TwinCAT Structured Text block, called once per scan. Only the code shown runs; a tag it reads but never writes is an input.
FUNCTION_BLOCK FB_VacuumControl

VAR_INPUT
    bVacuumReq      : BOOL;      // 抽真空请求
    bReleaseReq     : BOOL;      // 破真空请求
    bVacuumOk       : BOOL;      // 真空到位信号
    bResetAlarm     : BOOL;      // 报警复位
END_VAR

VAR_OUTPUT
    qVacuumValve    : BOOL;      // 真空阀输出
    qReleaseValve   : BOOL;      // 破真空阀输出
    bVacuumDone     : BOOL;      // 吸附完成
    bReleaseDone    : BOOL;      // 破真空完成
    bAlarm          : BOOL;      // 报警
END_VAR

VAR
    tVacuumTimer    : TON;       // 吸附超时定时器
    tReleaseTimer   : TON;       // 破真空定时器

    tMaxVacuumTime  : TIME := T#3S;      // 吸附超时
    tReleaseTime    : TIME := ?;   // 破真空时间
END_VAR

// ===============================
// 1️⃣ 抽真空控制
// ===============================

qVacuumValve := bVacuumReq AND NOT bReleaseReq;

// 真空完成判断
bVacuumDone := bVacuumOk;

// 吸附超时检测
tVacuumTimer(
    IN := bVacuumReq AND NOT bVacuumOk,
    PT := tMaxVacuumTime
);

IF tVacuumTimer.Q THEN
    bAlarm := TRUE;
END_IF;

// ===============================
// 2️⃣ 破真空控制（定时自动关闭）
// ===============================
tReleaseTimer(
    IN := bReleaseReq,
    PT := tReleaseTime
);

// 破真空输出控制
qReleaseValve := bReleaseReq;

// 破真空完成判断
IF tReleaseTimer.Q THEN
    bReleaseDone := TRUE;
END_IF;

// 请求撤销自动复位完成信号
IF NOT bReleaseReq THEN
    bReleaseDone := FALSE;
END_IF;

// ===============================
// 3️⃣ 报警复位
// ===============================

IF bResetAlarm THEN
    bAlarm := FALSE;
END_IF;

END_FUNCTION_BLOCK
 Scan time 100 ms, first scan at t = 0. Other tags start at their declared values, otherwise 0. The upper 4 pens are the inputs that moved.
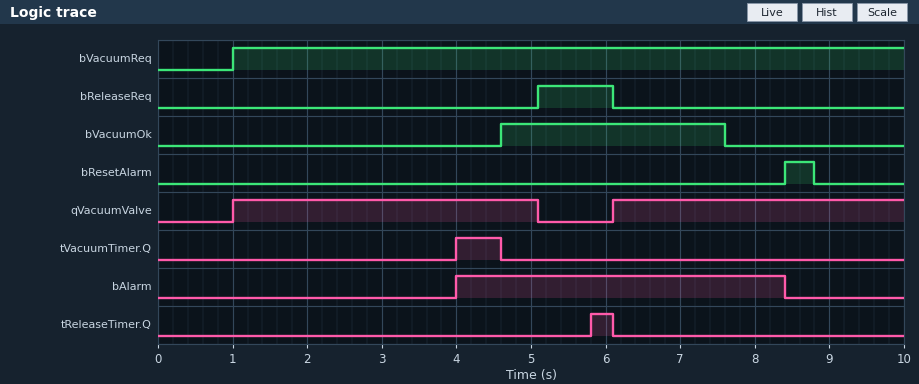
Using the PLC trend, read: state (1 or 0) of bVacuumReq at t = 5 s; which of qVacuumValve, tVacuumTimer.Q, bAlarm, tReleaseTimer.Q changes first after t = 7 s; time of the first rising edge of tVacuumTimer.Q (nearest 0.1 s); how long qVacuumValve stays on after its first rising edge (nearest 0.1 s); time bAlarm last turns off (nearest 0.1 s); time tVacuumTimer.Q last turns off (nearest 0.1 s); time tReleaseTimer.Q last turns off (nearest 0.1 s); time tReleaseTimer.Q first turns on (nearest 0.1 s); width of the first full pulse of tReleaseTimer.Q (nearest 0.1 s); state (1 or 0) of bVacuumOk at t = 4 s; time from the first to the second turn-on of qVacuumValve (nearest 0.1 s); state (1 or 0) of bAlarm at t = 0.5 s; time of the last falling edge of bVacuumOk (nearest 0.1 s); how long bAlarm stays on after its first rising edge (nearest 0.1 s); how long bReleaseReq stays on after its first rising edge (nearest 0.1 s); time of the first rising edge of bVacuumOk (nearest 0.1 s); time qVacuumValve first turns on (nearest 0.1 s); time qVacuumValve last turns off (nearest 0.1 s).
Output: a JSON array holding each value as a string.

["1", "bAlarm", "4.0 s", "4.1 s", "8.4 s", "4.6 s", "6.1 s", "5.8 s", "0.3 s", "0", "5.1 s", "0", "7.6 s", "4.4 s", "1.0 s", "4.6 s", "1.0 s", "5.1 s"]
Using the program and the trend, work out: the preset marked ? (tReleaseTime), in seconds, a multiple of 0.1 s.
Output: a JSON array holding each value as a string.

["0.7 s"]
